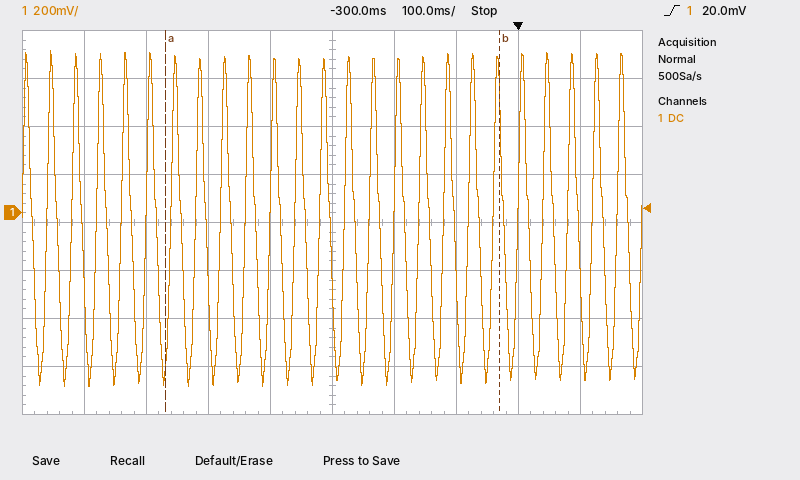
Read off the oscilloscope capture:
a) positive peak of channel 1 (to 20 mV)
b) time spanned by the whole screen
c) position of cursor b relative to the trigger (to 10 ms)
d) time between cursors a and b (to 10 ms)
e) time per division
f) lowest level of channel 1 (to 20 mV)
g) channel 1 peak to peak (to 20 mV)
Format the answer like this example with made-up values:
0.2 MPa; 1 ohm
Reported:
680 mV; 1 s; -30 ms; 540 ms; 100 ms; -720 mV; 1.40 V
